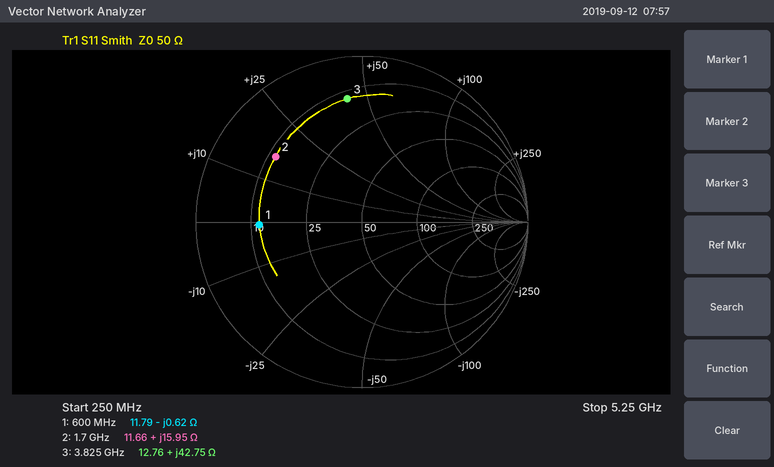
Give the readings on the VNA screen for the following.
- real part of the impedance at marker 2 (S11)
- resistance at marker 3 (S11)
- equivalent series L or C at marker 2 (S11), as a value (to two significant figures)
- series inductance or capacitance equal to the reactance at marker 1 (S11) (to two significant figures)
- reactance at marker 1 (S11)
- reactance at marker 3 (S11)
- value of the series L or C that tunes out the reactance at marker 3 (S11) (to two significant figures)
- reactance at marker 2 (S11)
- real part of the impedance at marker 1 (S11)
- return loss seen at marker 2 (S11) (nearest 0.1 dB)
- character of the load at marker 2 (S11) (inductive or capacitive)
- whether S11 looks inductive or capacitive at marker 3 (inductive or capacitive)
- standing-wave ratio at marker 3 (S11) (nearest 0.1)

11.66 Ω
12.76 Ω
1.5 nH
430 pF
-0.62 Ω
+42.75 Ω
970 fF
+15.95 Ω
11.79 Ω
3.7 dB
inductive
inductive
6.9
